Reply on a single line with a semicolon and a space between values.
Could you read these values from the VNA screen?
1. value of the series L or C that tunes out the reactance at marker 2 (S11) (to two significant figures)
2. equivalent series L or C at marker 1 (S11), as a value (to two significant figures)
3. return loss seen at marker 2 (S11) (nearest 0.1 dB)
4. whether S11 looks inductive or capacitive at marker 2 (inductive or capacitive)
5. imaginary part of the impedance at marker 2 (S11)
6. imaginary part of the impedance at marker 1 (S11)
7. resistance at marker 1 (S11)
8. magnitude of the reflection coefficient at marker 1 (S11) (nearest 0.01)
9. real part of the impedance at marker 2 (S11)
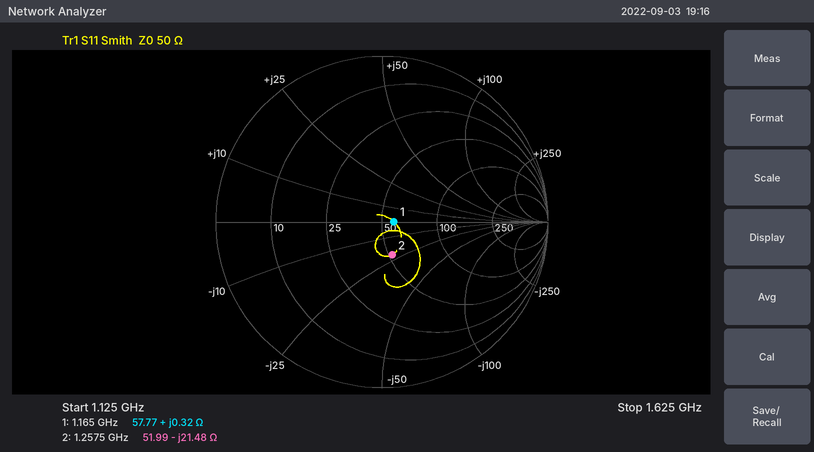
2.7 nH; 44 pH; 13.7 dB; capacitive; -21.48 Ω; +0.32 Ω; 57.77 Ω; 0.07; 51.99 Ω
